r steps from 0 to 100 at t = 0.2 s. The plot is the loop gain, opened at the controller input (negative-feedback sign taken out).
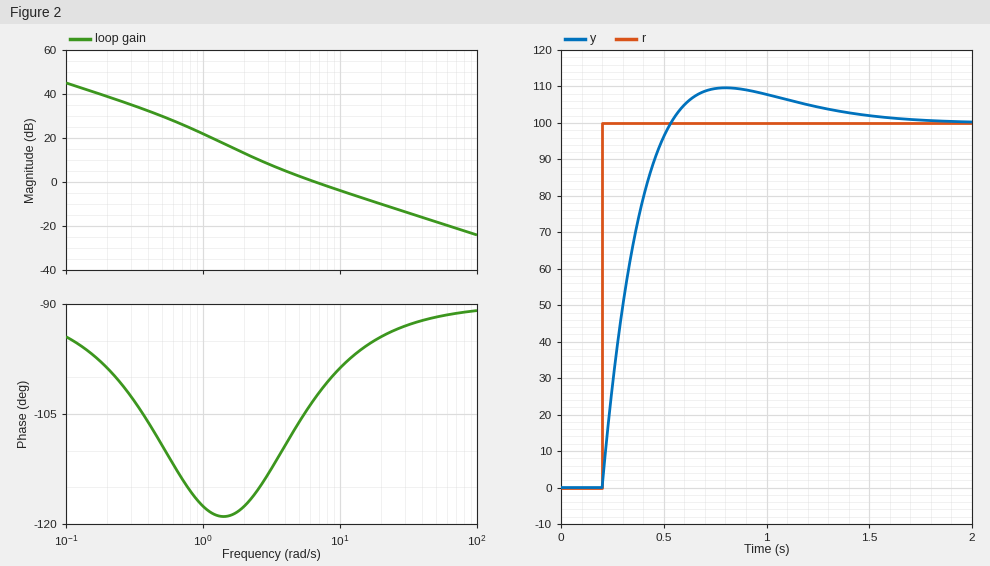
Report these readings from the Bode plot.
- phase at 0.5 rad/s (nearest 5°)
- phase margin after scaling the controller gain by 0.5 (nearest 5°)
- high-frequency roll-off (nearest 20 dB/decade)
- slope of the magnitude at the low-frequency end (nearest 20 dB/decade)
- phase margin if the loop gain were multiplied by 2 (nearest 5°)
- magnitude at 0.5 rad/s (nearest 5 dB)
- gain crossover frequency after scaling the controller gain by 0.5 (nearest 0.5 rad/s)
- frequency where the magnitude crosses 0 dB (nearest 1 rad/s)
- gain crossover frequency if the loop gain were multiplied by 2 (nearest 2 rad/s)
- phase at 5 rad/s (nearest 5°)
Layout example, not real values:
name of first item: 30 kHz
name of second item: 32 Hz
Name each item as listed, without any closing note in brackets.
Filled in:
phase at 0.5 rad/s: -110°
phase margin after scaling the controller gain by 0.5: 70°
high-frequency roll-off: -20 dB/decade
slope of the magnitude at the low-frequency end: -20 dB/decade
phase margin if the loop gain were multiplied by 2: 85°
magnitude at 0.5 rad/s: 30 dB
gain crossover frequency after scaling the controller gain by 0.5: 3.5 rad/s
frequency where the magnitude crosses 0 dB: 7 rad/s
gain crossover frequency if the loop gain were multiplied by 2: 12 rad/s
phase at 5 rad/s: -105°
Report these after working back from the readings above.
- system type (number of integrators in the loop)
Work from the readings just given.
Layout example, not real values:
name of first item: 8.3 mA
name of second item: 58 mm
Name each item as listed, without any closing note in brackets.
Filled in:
system type: 1
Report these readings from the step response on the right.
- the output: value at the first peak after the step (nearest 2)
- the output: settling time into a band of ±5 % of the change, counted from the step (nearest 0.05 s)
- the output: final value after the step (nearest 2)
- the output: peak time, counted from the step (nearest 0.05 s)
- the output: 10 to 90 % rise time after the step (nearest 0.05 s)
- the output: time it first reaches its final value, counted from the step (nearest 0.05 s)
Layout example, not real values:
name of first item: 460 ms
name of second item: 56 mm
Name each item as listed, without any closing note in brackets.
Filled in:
the output: value at the first peak after the step: 110
the output: settling time into a band of ±5 % of the change, counted from the step: 1.00 s
the output: final value after the step: 100
the output: peak time, counted from the step: 0.60 s
the output: 10 to 90 % rise time after the step: 0.25 s
the output: time it first reaches its final value, counted from the step: 0.35 s
